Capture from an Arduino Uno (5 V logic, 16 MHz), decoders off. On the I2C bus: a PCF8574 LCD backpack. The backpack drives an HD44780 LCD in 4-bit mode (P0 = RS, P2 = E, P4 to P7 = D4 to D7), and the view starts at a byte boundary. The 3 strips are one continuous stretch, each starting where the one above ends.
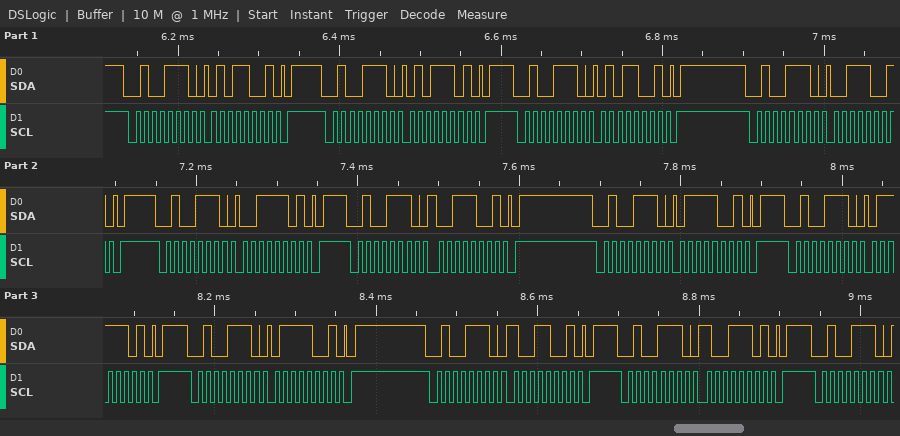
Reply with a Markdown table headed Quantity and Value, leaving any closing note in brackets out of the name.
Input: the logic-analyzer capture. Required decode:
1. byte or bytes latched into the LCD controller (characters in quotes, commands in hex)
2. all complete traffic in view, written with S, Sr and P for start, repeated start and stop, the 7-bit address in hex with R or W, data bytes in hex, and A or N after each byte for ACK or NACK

| Quantity | Value |
|---|---|
| byte or bytes latched into the LCD controller | 'S' |
| all complete traffic in view, written with S, Sr and P for start, repeated start and stop, the 7-bit address in hex with R or W, data bytes in hex, and A or N after each byte for ACK or NACK | S 27W A 59 A P S 27W A 5D A P S 27W A 59 A P S 27W A 39 A P S 27W A 3D A P S 27W A 39 A P S 27W A 79 A P S 27W A 7D A P S 27W A 79 A P S 27W A 99 A P S 27W A 9D A P S 27W A |
